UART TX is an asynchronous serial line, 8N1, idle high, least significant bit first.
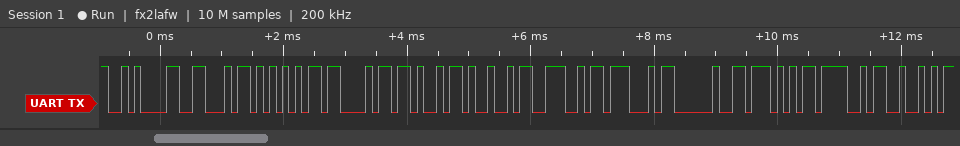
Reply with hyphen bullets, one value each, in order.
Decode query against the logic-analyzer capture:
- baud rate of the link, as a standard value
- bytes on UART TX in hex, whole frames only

- 9600 baud
- 0x0A 0x46 0x55 0x43 0x4B 0x49 0x4E 0x47 0x20 0x57 0x4F 0x52
